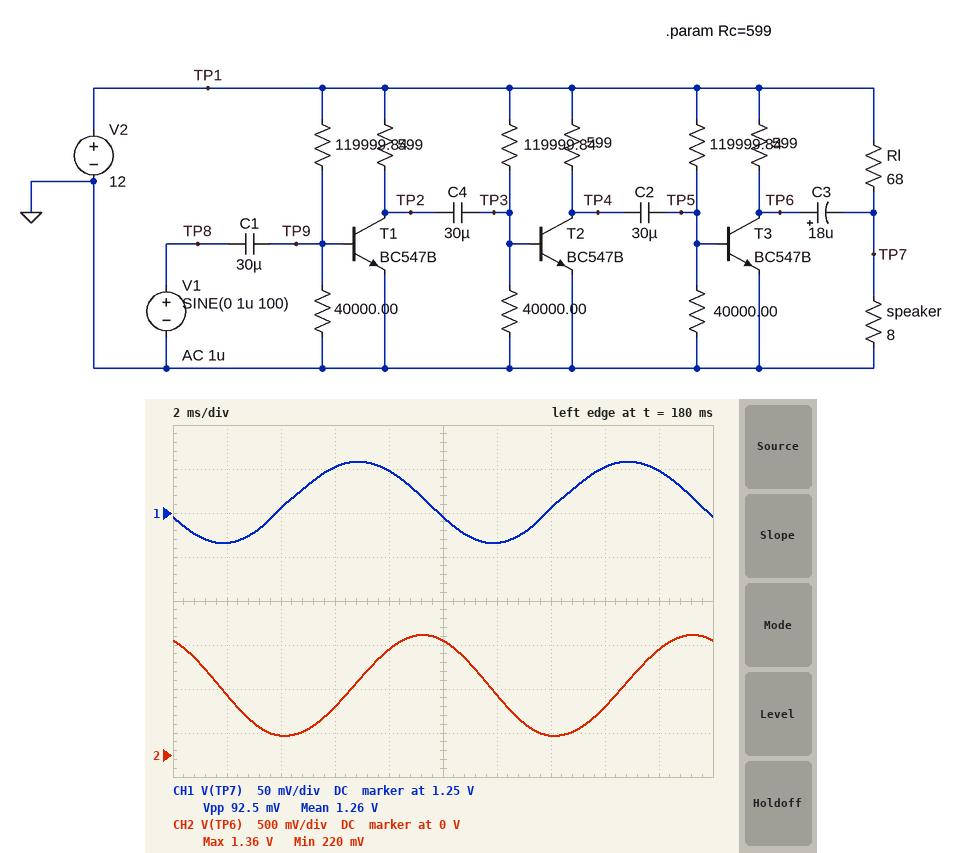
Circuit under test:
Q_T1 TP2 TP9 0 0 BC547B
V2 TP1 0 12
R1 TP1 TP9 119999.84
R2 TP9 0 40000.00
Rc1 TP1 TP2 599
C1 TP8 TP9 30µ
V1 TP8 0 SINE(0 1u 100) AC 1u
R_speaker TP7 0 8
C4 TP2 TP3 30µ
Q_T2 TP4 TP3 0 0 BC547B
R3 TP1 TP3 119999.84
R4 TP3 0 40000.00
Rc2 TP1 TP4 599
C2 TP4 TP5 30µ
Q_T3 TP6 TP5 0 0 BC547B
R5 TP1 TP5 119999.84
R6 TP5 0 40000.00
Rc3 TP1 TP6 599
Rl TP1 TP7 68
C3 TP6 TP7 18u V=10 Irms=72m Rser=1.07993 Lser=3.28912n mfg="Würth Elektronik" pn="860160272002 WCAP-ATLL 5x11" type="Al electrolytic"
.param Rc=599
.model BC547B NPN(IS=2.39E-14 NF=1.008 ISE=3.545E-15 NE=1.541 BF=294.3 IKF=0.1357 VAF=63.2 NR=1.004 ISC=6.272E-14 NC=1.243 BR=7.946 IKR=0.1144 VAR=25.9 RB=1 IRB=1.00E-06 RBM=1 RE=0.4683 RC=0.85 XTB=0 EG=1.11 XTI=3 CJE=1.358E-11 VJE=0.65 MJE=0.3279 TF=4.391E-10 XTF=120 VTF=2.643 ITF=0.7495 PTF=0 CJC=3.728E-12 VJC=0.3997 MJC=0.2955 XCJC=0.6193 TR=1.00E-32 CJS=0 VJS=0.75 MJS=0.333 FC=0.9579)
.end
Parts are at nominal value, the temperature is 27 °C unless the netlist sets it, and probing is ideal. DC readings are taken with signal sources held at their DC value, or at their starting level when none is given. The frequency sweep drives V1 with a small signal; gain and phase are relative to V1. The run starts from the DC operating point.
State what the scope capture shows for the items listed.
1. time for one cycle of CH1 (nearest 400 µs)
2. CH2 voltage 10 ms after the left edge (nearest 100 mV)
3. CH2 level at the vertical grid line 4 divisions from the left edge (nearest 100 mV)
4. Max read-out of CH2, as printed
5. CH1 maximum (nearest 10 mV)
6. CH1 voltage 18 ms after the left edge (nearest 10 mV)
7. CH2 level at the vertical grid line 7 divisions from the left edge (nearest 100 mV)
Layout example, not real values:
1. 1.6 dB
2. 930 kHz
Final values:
1. 10.0 ms
2. 1.3 V
3. 1.2 V
4. 1.36 V
5. 1.31 V
6. 1.30 V
7. 200 mV
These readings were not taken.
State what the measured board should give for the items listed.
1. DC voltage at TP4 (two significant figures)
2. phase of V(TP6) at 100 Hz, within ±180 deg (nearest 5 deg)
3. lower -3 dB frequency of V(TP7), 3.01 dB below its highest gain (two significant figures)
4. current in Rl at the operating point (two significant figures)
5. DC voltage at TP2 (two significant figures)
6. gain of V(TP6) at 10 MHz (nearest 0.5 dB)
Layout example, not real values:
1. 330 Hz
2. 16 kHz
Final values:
1. 690 mV
2. 120 deg
3. 25 Hz
4. 160 mA
5. 690 mV
6. 64.0 dB
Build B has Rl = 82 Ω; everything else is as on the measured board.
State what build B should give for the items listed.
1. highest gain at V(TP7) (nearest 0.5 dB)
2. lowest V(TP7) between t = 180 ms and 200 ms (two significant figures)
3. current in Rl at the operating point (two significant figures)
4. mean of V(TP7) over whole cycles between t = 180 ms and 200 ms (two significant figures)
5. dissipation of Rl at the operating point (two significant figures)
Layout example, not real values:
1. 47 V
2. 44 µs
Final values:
1. 94.0 dB
2. 1.0 V
3. 130 mA
4. 1.1 V
5. 1.5 W
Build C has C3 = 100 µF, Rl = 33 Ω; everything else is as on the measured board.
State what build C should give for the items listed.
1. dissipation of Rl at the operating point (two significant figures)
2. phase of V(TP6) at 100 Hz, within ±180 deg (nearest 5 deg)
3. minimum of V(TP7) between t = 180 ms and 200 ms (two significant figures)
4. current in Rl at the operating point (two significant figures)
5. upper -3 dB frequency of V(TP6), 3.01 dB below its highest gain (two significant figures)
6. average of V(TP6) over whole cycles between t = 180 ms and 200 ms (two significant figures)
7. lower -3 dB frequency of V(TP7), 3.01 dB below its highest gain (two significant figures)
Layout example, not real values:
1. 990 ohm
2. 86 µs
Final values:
1. 2.8 W
2. 130 deg
3. 2.3 V
4. 290 mA
5. 26 Hz
6. 750 mV
7. 16 Hz
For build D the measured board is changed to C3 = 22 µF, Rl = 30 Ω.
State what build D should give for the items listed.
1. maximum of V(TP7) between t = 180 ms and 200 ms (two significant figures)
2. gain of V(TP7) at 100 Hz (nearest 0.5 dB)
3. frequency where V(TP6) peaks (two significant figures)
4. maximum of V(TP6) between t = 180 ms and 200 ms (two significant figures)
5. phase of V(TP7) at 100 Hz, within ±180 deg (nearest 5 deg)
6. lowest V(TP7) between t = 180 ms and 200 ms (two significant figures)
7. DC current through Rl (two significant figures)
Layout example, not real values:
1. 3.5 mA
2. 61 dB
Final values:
1. 2.6 V
2. 92.5 dB
3. 16 Hz
4. 1.2 V
5. -160 deg
6. 2.5 V
7. 320 mA
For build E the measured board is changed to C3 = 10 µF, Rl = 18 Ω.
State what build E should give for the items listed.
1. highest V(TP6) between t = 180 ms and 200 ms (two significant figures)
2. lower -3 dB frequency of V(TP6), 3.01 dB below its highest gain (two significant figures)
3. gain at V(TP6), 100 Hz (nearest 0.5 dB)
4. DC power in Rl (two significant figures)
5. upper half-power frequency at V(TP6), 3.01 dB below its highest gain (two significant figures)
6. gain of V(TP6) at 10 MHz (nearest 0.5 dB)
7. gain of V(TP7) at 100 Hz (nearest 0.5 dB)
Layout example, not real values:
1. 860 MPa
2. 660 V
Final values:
1. 2.0 V
2. 10 Hz
3. 120.0 dB
4. 3.8 W
5. 54 Hz
6. 62.0 dB
7. 91.0 dB
